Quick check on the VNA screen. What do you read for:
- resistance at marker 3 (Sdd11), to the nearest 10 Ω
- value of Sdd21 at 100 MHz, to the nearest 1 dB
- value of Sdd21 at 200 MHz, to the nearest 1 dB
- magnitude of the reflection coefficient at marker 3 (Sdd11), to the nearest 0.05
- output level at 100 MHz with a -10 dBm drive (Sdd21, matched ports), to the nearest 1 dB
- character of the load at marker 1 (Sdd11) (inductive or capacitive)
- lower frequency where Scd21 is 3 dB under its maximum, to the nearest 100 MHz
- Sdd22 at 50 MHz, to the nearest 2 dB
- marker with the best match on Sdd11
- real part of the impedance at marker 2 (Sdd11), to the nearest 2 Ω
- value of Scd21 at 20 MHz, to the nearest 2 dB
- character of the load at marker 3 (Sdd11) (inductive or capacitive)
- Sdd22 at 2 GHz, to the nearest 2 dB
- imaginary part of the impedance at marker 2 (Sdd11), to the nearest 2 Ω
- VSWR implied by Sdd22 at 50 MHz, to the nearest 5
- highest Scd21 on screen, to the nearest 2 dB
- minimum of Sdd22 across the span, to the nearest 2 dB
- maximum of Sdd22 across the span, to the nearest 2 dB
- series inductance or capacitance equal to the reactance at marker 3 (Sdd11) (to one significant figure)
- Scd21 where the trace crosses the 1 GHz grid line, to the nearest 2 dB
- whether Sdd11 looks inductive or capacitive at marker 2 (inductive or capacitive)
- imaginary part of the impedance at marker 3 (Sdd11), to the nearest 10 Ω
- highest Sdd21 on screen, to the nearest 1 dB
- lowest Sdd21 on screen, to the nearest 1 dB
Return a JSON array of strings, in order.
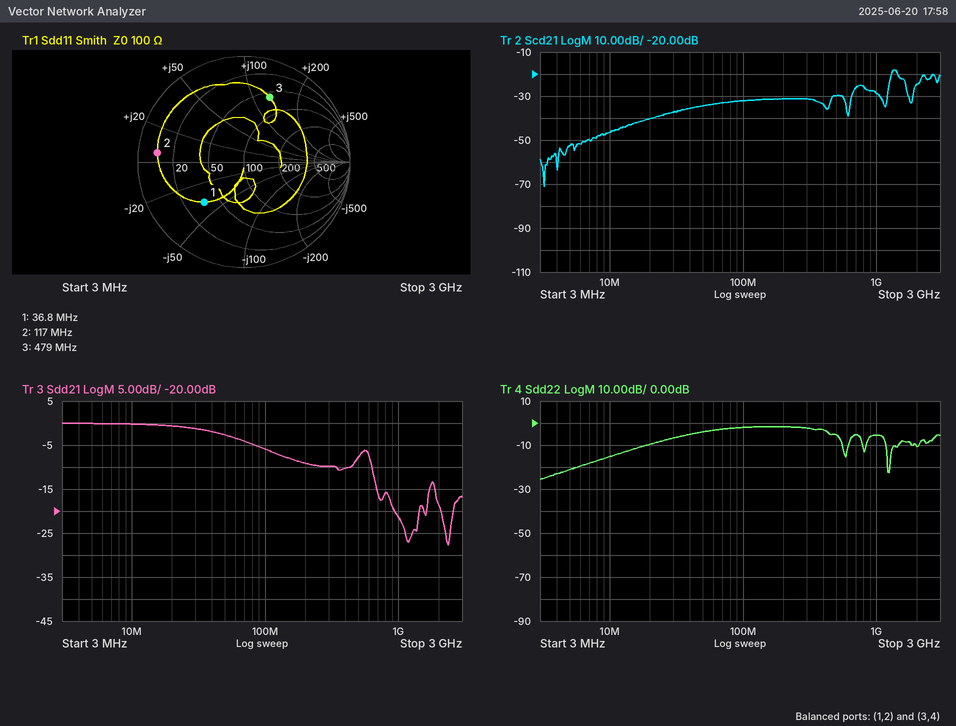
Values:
["60 Ω", "-6 dB", "-9 dB", "0.65", "-16 dBm", "capacitive", "1.3 GHz", "-4 dB", "marker 1", "10 Ω", "-40 dB", "inductive", "-10 dB", "+6 Ω", "5", "-18 dB", "-26 dB", "-2 dB", "40 nH", "-28 dB", "inductive", "+130 Ω", "0 dB", "-28 dB"]
